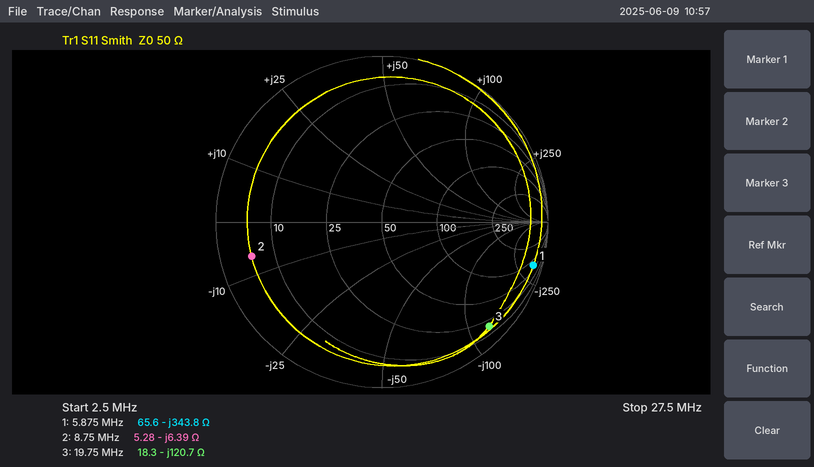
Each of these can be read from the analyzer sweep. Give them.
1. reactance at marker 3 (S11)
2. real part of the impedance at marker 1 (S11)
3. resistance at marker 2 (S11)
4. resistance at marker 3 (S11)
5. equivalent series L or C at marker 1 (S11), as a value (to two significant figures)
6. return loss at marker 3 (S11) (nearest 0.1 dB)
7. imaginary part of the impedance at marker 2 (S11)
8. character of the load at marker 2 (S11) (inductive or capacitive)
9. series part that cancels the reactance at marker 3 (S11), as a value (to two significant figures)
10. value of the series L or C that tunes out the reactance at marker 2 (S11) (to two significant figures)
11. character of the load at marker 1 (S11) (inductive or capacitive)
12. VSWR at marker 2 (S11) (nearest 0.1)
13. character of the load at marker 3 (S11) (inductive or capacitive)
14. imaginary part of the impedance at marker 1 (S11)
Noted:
-120.7 Ω
65.6 Ω
5.28 Ω
18.3 Ω
79 pF
0.9 dB
-6.39 Ω
capacitive
970 nH
120 nH
capacitive
9.6
capacitive
-343.8 Ω
